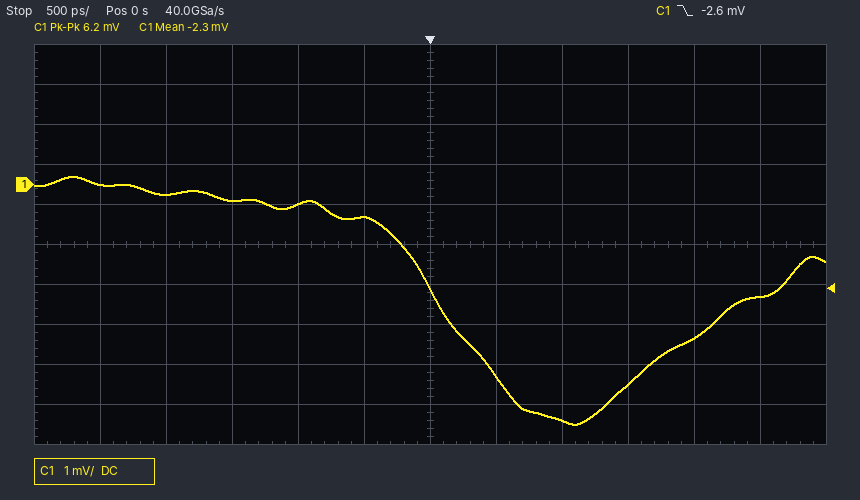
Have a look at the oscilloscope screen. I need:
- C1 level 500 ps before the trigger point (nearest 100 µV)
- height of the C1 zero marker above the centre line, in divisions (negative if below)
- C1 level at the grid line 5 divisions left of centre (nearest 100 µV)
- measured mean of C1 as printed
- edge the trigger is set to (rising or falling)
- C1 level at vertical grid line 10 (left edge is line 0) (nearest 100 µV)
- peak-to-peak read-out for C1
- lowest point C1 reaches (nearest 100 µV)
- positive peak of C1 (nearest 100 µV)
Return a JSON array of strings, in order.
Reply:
["-800 µV", "+1.5 div", "0.0 mV", "-2.3 mV", "falling", "-3.8 mV", "6.2 mV", "-6.0 mV", "200 µV"]
